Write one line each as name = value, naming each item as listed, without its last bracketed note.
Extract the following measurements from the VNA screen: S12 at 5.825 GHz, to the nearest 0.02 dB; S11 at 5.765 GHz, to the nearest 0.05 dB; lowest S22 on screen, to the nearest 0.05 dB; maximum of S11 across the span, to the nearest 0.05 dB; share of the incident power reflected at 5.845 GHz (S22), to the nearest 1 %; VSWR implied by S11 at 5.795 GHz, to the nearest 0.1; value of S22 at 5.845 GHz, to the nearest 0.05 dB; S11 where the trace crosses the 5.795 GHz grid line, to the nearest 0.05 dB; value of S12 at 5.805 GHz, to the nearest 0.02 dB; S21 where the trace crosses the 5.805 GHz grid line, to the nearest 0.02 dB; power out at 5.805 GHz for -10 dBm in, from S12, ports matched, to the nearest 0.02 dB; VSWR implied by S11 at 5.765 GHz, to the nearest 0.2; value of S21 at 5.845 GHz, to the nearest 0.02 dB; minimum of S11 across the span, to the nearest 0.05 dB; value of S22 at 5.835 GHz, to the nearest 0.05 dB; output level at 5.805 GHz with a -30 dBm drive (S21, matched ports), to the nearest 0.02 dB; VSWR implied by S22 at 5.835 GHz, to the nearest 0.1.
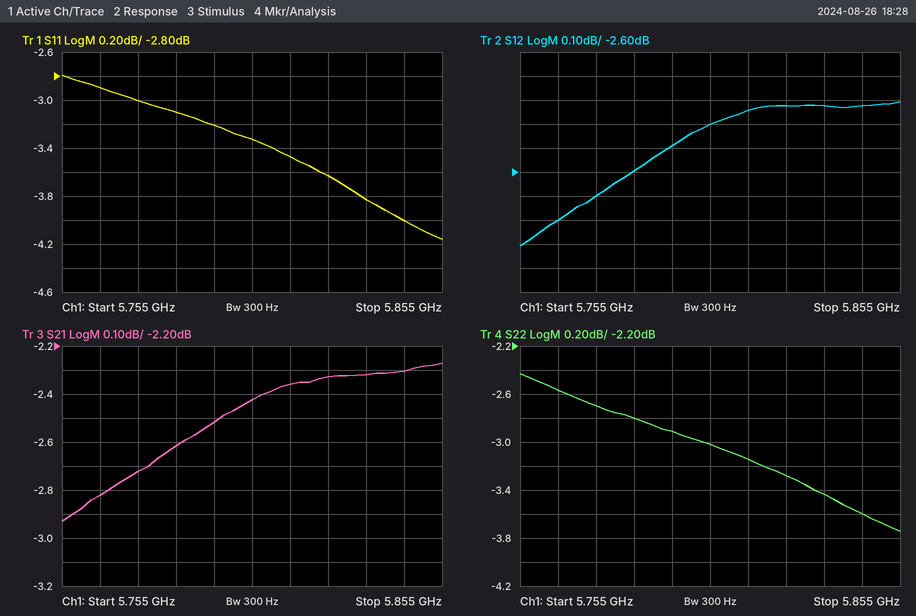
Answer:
S12 at 5.825 GHz, to the nearest 0.02 dB = -2.32 dB
S11 at 5.765 GHz, to the nearest 0.05 dB = -2.90 dB
lowest S22 on screen, to the nearest 0.05 dB = -3.75 dB
maximum of S11 across the span, to the nearest 0.05 dB = -2.80 dB
share of the incident power reflected at 5.845 GHz (S22), to the nearest 1 % = 44 %
VSWR implied by S11 at 5.795 GHz, to the nearest 0.1 = 5.5
value of S22 at 5.845 GHz, to the nearest 0.05 dB = -3.60 dB
S11 where the trace crosses the 5.795 GHz grid line, to the nearest 0.05 dB = -3.20 dB
value of S12 at 5.805 GHz, to the nearest 0.02 dB = -2.40 dB
S21 where the trace crosses the 5.805 GHz grid line, to the nearest 0.02 dB = -2.42 dB
power out at 5.805 GHz for -10 dBm in, from S12, ports matched, to the nearest 0.02 dB = -12.40 dBm
VSWR implied by S11 at 5.765 GHz, to the nearest 0.2 = 6.0
value of S21 at 5.845 GHz, to the nearest 0.02 dB = -2.30 dB
minimum of S11 across the span, to the nearest 0.05 dB = -4.15 dB
value of S22 at 5.835 GHz, to the nearest 0.05 dB = -3.45 dB
output level at 5.805 GHz with a -30 dBm drive (S21, matched ports), to the nearest 0.02 dB = -32.42 dBm
VSWR implied by S22 at 5.835 GHz, to the nearest 0.1 = 5.1
